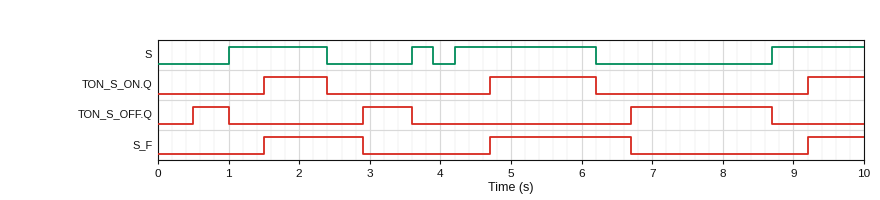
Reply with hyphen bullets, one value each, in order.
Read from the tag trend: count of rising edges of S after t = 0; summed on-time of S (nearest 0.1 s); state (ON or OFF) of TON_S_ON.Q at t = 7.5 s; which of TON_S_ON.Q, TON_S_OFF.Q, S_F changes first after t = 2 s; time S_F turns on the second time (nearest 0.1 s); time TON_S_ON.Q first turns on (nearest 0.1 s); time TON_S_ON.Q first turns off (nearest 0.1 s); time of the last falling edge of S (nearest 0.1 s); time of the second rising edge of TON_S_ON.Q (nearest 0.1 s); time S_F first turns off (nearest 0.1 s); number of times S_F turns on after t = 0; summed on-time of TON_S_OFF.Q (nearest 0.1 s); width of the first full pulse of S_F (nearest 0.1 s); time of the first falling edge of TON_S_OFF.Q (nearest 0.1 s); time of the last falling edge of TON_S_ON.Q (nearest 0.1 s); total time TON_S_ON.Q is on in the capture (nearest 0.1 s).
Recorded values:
- 4
- 5.0 s
- OFF
- TON_S_ON.Q
- 4.7 s
- 1.5 s
- 2.4 s
- 6.2 s
- 4.7 s
- 2.9 s
- 3
- 3.2 s
- 1.4 s
- 1.0 s
- 6.2 s
- 3.2 s
